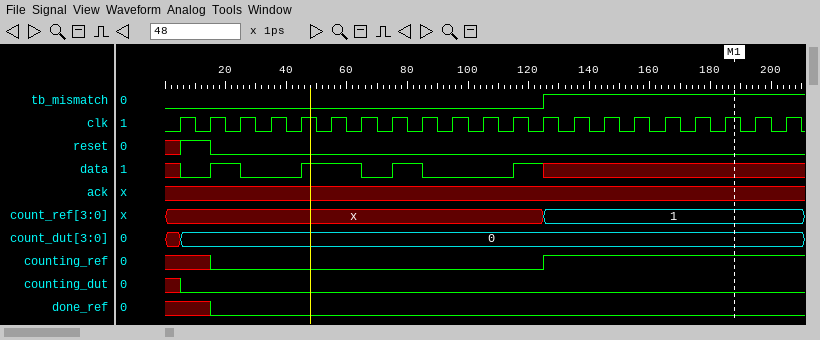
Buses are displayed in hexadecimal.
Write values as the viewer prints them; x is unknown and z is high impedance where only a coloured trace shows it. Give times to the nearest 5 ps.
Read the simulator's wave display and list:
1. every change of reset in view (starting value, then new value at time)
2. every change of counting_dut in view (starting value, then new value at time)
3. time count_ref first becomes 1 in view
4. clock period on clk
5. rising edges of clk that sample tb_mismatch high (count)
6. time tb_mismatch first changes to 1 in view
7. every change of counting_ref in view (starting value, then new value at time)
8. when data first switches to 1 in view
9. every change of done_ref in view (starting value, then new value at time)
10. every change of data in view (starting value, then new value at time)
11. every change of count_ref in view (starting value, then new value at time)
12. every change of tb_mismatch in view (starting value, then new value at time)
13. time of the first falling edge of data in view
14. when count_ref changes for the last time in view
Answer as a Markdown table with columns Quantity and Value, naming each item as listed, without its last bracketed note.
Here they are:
| Quantity | Value |
|---|---|
| every change of reset in view | x, 1 at 5 ps, 0 at 15 ps |
| every change of counting_dut in view | x, 0 at 5 ps |
| time count_ref first becomes 1 in view | 125 ps |
| clock period on clk | 10 ps |
| rising edges of clk that sample tb_mismatch high | 8 |
| time tb_mismatch first changes to 1 in view | 125 ps |
| every change of counting_ref in view | x, 0 at 15 ps, 1 at 125 ps |
| when data first switches to 1 in view | 15 ps |
| every change of done_ref in view | x, 0 at 15 ps |
| every change of data in view | x, 0 at 5 ps, 1 at 15 ps, 0 at 25 ps, 1 at 45 ps, 0 at 65 ps, 1 at 75 ps, 0 at 85 ps, 1 at 115 ps, x at 125 ps |
| every change of count_ref in view | x, 1 at 125 ps |
| every change of tb_mismatch in view | 0, 1 at 125 ps |
| time of the first falling edge of data in view | 25 ps |
| when count_ref changes for the last time in view | 125 ps |
